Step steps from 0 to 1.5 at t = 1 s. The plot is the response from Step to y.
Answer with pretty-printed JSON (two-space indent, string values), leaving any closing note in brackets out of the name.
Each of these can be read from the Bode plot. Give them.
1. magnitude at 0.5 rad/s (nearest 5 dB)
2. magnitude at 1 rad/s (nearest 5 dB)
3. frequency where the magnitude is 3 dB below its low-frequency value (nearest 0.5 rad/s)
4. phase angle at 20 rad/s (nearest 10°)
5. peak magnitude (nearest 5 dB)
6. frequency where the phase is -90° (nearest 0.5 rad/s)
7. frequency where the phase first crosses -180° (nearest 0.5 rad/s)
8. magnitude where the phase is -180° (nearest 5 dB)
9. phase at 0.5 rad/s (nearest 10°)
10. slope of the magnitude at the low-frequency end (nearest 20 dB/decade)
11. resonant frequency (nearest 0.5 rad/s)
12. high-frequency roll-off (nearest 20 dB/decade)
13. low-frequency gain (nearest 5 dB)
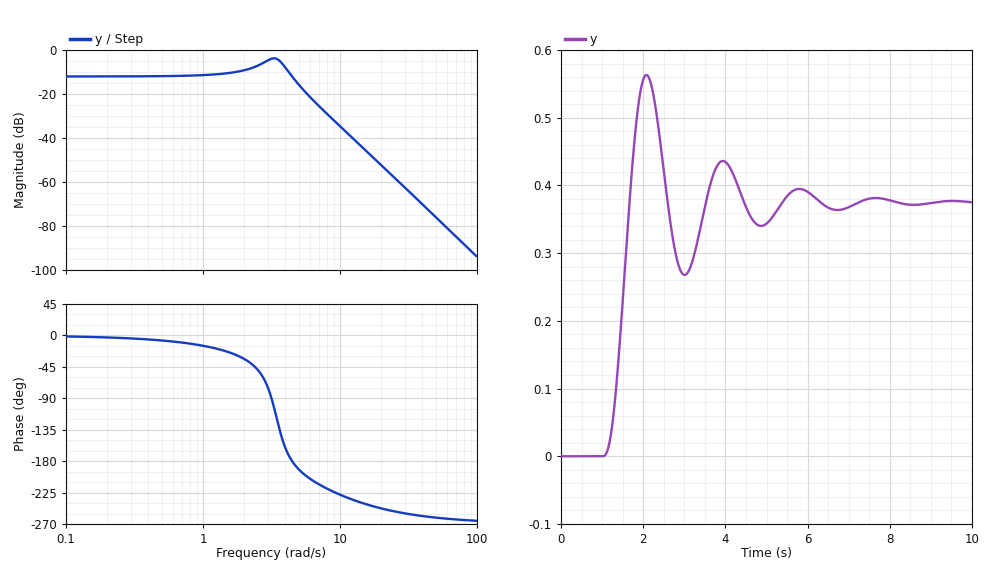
{
  "magnitude at 0.5 rad/s": "-10 dB",
  "magnitude at 1 rad/s": "-10 dB",
  "frequency where the magnitude is 3 dB below its low-frequency value": "5.0 rad/s",
  "phase angle at 20 rad/s": "-250°",
  "peak magnitude": "-5 dB",
  "frequency where the phase is -90°": "3.0 rad/s",
  "frequency where the phase first crosses -180°": "4.5 rad/s",
  "magnitude where the phase is -180°": "-10 dB",
  "phase at 0.5 rad/s": "-10°",
  "slope of the magnitude at the low-frequency end": "0 dB/decade",
  "resonant frequency": "3.5 rad/s",
  "high-frequency roll-off": "-60 dB/decade",
  "low-frequency gain": "-10 dB"
}
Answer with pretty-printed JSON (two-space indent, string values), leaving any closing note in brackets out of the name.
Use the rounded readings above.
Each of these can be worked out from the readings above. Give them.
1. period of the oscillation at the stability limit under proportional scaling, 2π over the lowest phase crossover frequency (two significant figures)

{
  "period of the oscillation at the stability limit under proportional scaling, 2π over the lowest phase crossover frequency": "1.4 s"
}
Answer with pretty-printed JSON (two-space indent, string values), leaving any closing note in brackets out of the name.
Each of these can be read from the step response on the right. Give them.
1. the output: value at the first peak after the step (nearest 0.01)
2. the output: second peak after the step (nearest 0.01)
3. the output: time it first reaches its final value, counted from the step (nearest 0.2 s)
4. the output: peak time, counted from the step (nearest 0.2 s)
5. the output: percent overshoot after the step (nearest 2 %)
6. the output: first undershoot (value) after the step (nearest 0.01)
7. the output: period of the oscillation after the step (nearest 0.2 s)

{
  "the output: value at the first peak after the step": "0.56",
  "the output: second peak after the step": "0.44",
  "the output: time it first reaches its final value, counted from the step": "0.6 s",
  "the output: peak time, counted from the step": "1.0 s",
  "the output: percent overshoot after the step": "50 %",
  "the output: first undershoot (value) after the step": "0.27",
  "the output: period of the oscillation after the step": "1.8 s"
}
